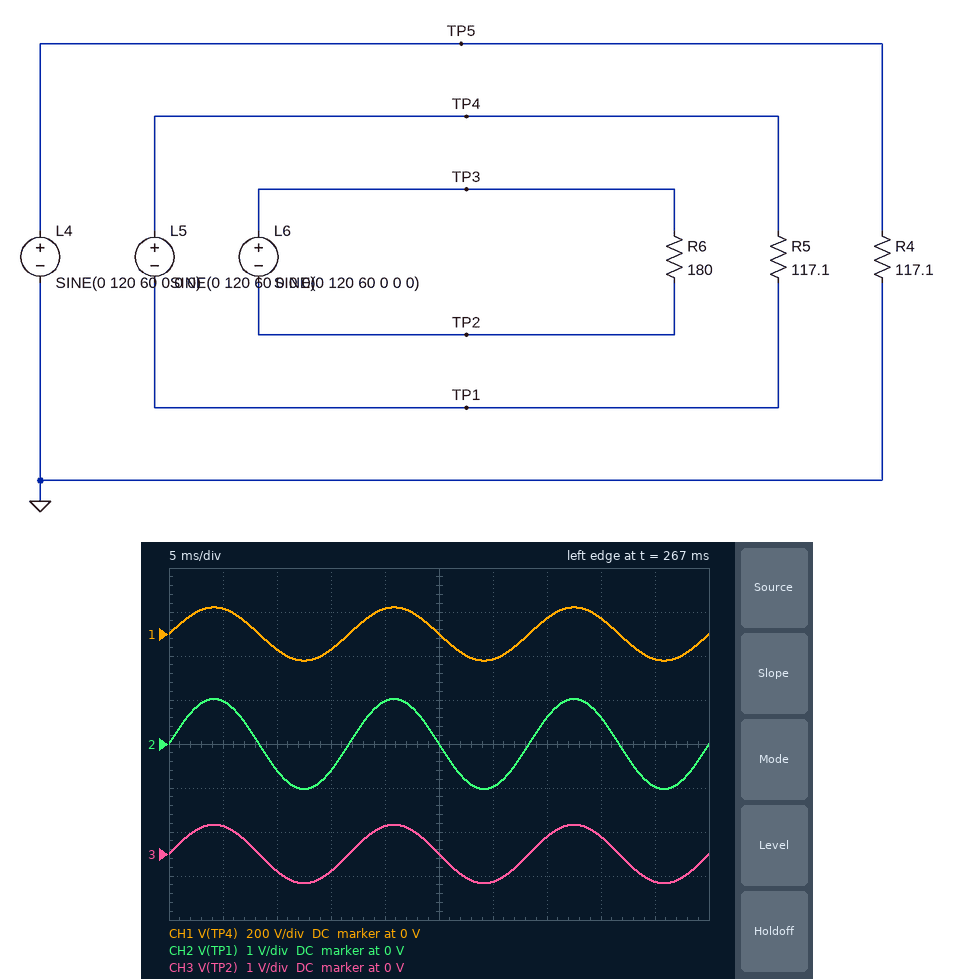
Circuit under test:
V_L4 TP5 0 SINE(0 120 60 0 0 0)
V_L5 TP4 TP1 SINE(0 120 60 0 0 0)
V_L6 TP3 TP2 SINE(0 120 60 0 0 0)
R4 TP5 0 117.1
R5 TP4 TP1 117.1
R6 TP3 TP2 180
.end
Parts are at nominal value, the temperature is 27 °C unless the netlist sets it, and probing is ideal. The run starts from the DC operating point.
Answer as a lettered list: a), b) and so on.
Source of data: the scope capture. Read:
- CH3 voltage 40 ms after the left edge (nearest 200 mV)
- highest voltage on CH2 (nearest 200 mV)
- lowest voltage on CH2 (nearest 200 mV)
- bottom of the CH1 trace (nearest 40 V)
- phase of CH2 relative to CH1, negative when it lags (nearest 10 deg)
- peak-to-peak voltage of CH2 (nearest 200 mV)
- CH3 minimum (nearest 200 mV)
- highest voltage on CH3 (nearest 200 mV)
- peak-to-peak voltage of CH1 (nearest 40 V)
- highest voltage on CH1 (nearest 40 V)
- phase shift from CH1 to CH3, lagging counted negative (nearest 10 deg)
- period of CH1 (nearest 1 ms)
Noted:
a) 400 mV
b) 1.0 V
c) -1.0 V
d) -120 V
e) 0 deg
f) 2.0 V
g) -600 mV
h) 600 mV
i) 240 V
j) 120 V
k) 0 deg
l) 17 ms
